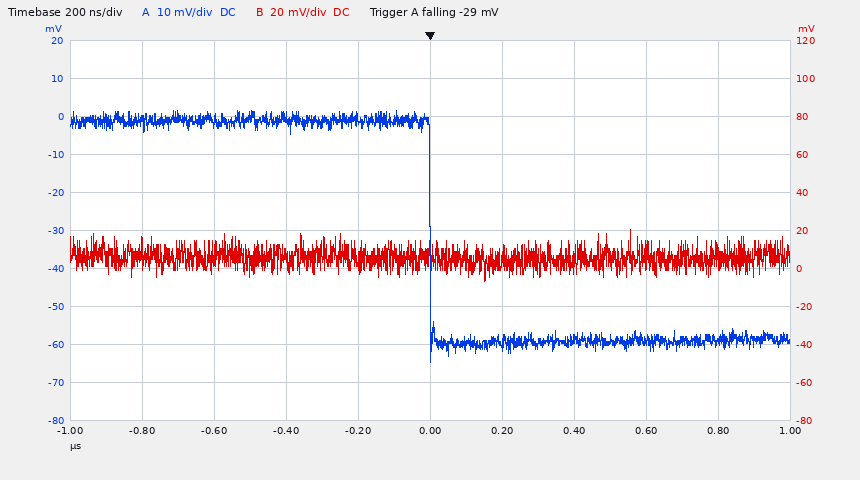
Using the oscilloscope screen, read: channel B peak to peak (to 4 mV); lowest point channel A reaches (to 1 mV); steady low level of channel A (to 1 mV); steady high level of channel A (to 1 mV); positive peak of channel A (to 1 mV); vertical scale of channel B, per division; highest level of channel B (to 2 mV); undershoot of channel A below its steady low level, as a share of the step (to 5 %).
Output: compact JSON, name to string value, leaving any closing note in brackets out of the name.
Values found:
{"channel B peak to peak": "28 mV", "lowest point channel A reaches": "-65 mV", "steady low level of channel A": "-59 mV", "steady high level of channel A": "-1 mV", "positive peak of channel A": "2 mV", "vertical scale of channel B, per division": "20 mV", "highest level of channel B": "20 mV", "undershoot of channel A below its steady low level, as a share of the step": "10 %"}
